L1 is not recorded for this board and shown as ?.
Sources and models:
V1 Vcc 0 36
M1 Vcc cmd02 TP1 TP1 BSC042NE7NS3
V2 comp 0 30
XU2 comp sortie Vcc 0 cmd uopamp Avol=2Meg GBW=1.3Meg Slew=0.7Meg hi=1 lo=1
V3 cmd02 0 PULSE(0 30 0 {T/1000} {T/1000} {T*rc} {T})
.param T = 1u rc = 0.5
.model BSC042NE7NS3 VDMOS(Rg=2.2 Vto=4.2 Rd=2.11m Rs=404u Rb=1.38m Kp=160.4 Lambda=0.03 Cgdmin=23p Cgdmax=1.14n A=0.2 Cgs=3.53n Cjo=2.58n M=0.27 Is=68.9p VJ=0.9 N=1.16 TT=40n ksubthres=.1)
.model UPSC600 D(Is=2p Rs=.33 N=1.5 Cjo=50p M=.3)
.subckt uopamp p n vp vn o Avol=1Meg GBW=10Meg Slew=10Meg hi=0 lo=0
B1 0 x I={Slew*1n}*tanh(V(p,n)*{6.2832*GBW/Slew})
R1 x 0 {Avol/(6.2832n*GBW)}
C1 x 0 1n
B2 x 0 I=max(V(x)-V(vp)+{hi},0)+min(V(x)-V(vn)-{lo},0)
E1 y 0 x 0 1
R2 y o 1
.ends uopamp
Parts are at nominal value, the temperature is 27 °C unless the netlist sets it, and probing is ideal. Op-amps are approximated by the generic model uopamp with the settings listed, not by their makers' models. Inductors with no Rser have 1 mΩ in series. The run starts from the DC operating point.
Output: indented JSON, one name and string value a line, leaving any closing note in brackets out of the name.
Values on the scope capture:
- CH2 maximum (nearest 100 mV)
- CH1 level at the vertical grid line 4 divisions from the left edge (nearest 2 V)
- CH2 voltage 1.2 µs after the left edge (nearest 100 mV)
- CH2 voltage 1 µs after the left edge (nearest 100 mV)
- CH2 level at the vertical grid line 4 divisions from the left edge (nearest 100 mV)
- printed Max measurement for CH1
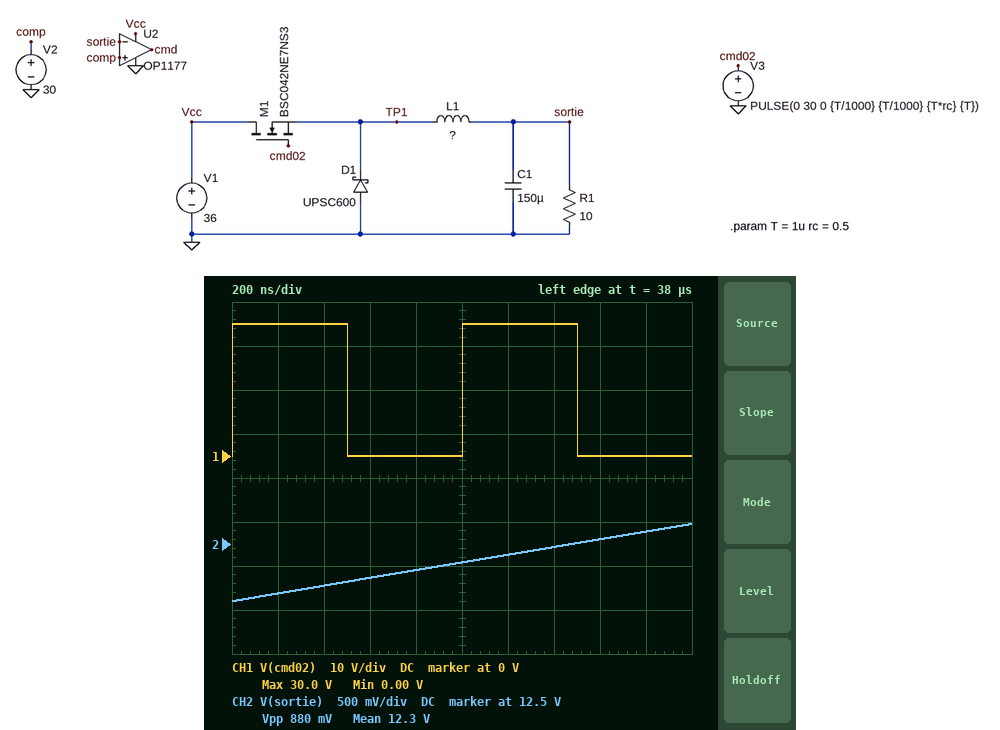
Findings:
{
  "CH2 maximum": "12.7 V",
  "CH1 level at the vertical grid line 4 divisions from the left edge": "0 V",
  "CH2 voltage 1.2 µs after the left edge": "12.4 V",
  "CH2 voltage 1 µs after the left edge": "12.3 V",
  "CH2 level at the vertical grid line 4 divisions from the left edge": "12.2 V",
  "printed Max measurement for CH1": "30.0 V"
}
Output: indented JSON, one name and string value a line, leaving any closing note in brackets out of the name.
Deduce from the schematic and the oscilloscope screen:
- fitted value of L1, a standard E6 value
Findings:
{
  "fitted value of L1, a standard E6 value": "3.3 µH"
}
